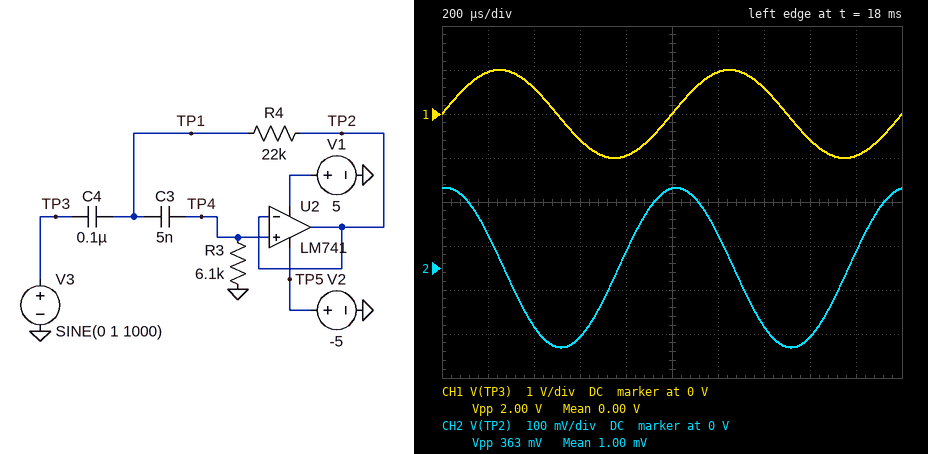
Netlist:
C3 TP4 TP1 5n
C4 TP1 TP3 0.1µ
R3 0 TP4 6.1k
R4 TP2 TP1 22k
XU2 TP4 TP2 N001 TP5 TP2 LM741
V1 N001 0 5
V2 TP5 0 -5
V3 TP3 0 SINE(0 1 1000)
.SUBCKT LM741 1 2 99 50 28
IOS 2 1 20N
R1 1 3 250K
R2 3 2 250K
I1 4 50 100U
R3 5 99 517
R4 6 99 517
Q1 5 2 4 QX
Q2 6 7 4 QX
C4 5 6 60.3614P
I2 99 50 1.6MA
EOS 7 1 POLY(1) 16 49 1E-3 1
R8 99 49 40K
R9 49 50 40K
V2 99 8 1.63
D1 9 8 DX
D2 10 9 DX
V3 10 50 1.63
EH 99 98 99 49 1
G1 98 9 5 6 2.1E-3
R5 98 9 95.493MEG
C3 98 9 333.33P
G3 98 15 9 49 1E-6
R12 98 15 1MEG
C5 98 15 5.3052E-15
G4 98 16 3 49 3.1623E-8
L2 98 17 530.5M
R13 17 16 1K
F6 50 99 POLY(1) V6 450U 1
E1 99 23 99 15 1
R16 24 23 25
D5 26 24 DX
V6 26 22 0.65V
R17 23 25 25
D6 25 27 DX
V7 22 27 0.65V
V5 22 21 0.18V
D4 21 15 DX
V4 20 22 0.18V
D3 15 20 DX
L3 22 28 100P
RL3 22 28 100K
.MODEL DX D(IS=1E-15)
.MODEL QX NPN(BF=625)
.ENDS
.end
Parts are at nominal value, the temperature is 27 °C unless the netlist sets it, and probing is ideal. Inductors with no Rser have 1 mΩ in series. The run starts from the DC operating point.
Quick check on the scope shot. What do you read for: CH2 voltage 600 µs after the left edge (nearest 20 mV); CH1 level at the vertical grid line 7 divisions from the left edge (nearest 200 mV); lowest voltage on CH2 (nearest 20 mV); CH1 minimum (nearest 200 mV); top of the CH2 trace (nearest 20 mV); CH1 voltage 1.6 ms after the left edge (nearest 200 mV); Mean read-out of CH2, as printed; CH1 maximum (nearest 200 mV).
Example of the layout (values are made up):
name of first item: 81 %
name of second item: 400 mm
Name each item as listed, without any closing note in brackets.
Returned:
CH2 voltage 600 µs after the left edge: -160 mV
CH1 level at the vertical grid line 7 divisions from the left edge: 600 mV
lowest voltage on CH2: -180 mV
CH1 minimum: -1.0 V
top of the CH2 trace: 180 mV
CH1 voltage 1.6 ms after the left edge: -600 mV
Mean read-out of CH2, as printed: 1.00 mV
CH1 maximum: 1.0 V
